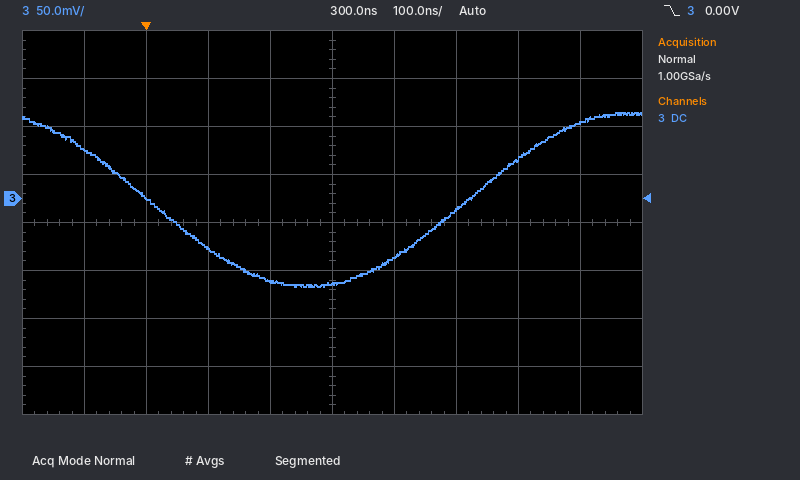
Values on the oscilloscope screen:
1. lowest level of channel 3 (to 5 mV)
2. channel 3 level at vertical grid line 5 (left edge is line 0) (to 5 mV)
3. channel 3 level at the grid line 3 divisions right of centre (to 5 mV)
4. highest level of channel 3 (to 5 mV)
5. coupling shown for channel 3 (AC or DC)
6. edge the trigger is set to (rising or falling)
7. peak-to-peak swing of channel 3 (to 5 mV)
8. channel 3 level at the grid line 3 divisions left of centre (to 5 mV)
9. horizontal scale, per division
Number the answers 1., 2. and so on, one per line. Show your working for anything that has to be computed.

1. -90 mV
2. -90 mV
3. 40 mV
4. 90 mV
5. DC
6. falling
7. 90 mV − (-90 mV) = 180 mV
8. 0 mV
9. 100 ns
